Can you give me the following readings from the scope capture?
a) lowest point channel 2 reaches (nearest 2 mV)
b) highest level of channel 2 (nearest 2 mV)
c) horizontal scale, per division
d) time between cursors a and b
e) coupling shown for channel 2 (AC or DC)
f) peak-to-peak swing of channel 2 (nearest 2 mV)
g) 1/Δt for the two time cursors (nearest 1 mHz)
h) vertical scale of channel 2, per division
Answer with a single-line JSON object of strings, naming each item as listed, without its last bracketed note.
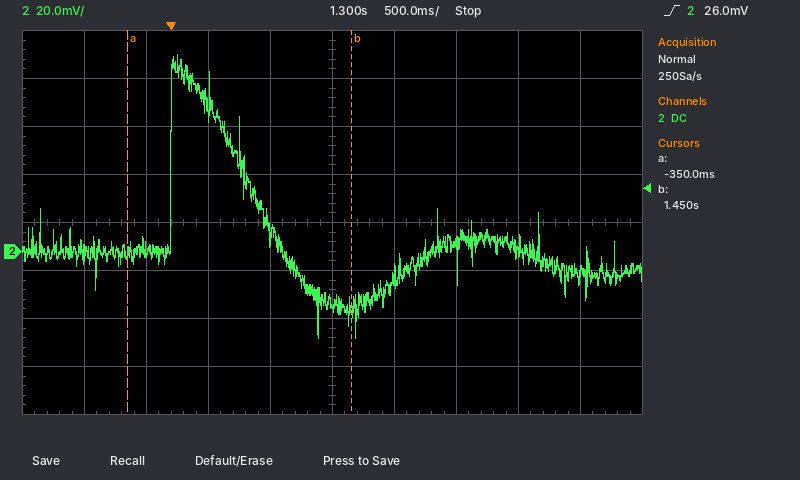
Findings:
{"lowest point channel 2 reaches": "-36 mV", "highest level of channel 2": "82 mV", "horizontal scale, per division": "500 ms", "time between cursors a and b": "1.80 s", "coupling shown for channel 2": "DC", "peak-to-peak swing of channel 2": "118 mV", "1/Δt for the two time cursors": "556 mHz", "vertical scale of channel 2, per division": "20 mV"}
